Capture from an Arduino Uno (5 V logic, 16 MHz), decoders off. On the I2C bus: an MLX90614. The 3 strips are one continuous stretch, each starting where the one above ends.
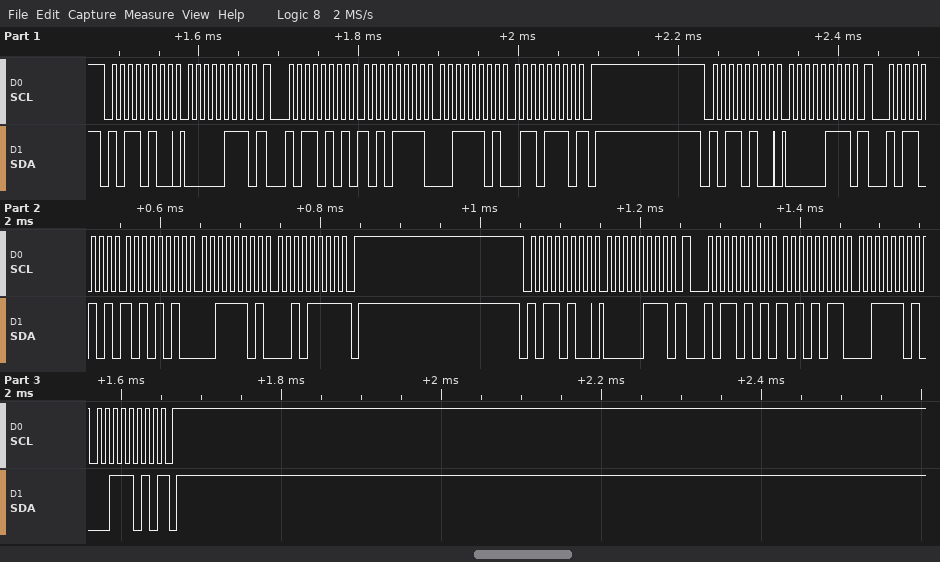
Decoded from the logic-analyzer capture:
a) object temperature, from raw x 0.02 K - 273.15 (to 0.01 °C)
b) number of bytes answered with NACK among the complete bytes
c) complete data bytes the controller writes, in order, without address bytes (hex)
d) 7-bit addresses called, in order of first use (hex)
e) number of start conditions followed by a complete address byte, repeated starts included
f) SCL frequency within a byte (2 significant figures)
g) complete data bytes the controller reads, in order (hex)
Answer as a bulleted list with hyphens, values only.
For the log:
- 42.67 °C
- 3
- 07 07 07
- 0x5A
- 6
- 100 kHz
- AF 3D 6E AA 3D 2F AB 3D 3A
